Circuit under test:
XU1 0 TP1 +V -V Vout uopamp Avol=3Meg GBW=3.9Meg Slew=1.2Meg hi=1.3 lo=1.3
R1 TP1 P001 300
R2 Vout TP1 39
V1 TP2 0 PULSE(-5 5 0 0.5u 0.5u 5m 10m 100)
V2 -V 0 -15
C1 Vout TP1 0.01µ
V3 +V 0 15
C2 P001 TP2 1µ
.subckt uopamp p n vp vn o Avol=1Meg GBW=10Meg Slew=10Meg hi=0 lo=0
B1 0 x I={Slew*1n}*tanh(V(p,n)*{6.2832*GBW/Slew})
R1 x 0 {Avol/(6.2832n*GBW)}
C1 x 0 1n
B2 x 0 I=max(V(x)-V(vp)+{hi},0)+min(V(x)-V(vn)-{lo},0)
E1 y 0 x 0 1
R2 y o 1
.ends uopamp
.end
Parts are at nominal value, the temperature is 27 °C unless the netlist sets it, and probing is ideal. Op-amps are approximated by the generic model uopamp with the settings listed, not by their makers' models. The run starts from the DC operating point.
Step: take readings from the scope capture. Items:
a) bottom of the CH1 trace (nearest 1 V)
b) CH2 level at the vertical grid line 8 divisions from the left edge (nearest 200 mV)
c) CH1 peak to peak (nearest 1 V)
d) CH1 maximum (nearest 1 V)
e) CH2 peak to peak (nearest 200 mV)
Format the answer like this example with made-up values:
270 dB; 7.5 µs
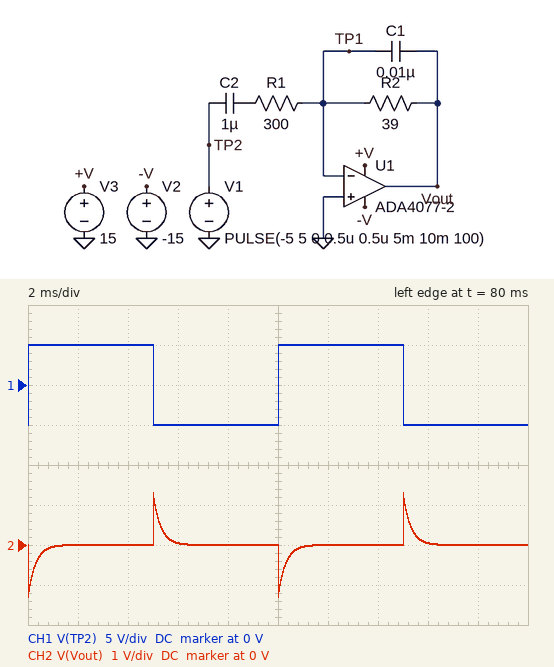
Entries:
-5 V; 0 V; 10 V; 5 V; 2.6 V
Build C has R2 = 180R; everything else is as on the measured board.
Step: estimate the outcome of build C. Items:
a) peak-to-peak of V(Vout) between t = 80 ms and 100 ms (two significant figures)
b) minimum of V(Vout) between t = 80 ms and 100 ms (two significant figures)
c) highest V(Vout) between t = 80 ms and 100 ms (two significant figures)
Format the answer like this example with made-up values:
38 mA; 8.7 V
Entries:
12 V; -5.8 V; 5.8 V
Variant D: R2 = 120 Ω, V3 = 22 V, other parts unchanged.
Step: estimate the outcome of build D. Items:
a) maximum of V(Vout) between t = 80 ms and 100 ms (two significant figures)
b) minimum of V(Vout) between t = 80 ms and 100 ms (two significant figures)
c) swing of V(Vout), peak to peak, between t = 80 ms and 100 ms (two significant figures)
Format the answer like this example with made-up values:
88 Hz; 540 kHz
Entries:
3.9 V; -3.9 V; 7.8 V
